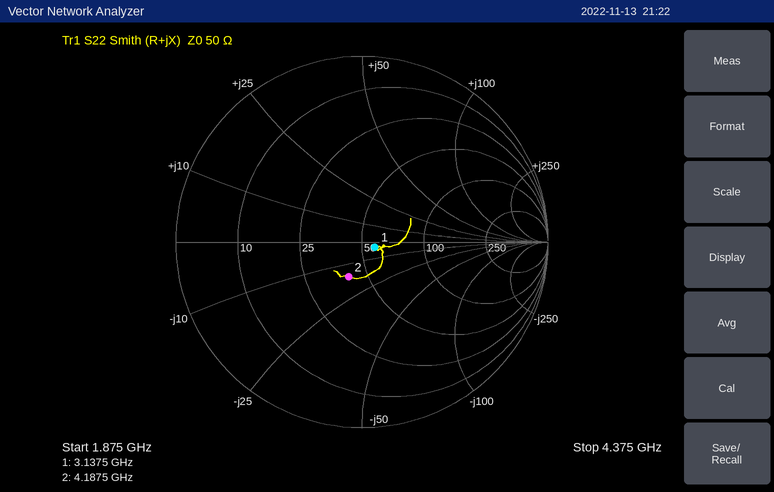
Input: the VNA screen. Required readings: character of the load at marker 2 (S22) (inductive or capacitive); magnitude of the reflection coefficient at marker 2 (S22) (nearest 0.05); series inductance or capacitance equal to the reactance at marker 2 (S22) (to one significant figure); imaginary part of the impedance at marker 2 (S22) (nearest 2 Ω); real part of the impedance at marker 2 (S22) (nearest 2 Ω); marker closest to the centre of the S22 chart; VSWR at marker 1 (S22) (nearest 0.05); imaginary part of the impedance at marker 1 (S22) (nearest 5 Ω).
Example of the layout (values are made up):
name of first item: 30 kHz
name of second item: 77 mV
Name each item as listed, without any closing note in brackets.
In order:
character of the load at marker 2 (S22): capacitive
magnitude of the reflection coefficient at marker 2 (S22): 0.20
series inductance or capacitance equal to the reactance at marker 2 (S22): 2 pF
imaginary part of the impedance at marker 2 (S22): -16 Ω
real part of the impedance at marker 2 (S22): 40 Ω
marker closest to the centre of the S22 chart: marker 1
VSWR at marker 1 (S22): 1.15
imaginary part of the impedance at marker 1 (S22): -5 Ω
